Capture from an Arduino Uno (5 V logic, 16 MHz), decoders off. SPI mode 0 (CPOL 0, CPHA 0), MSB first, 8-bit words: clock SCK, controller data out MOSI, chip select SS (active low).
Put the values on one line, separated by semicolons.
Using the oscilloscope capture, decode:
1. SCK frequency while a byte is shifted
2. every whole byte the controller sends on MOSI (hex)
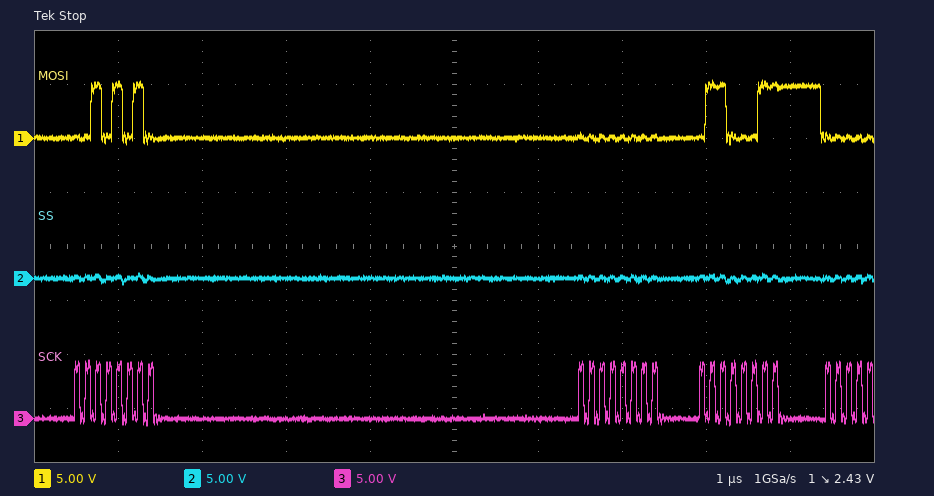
8 MHz; 2A 00 63
